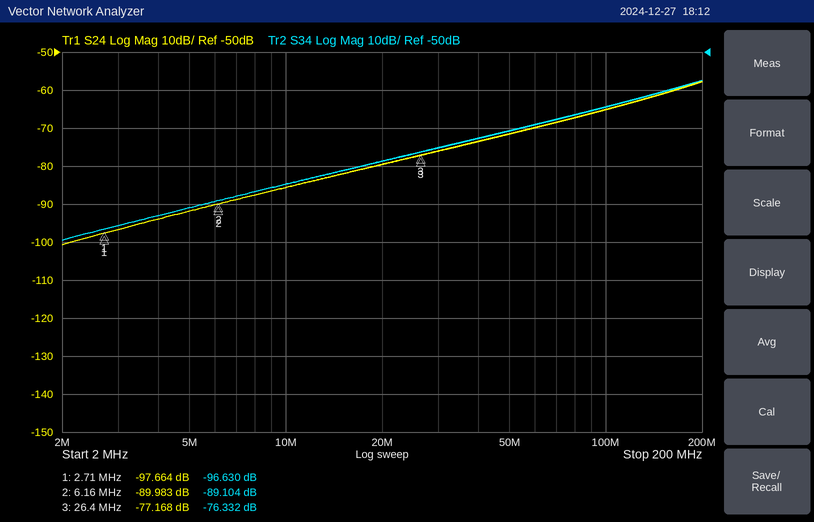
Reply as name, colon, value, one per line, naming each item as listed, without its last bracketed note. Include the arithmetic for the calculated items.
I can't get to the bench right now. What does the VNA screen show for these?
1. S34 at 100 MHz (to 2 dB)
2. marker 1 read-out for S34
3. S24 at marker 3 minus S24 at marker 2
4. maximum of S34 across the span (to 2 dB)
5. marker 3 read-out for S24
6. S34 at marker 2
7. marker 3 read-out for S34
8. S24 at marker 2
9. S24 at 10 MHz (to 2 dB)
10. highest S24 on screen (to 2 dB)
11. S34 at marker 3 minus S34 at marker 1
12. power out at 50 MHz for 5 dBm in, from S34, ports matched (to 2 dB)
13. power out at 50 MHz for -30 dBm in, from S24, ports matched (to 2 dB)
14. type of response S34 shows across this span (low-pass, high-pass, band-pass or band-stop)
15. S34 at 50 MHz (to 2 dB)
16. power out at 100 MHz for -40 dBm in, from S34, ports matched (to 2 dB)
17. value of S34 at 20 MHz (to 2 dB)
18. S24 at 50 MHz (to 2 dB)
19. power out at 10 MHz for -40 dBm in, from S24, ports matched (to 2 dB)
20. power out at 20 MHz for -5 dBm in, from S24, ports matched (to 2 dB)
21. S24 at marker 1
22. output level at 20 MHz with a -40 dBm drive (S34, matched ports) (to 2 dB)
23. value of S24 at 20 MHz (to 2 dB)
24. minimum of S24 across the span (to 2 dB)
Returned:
S34 at 100 MHz: -64 dB
marker 1 read-out for S34: -96.630 dB
S24 at marker 3 minus S24 at marker 2: -77.168 − (-89.983) = 12.815 dB
maximum of S34 across the span: -58 dB
marker 3 read-out for S24: -77.168 dB
S34 at marker 2: -89.104 dB
marker 3 read-out for S34: -76.332 dB
S24 at marker 2: -89.983 dB
S24 at 10 MHz: -86 dB
highest S24 on screen: -58 dB
S34 at marker 3 minus S34 at marker 1: -76.332 − (-96.63) = 20.298 dB
power out at 50 MHz for 5 dBm in, from S34, ports matched: 5 dBm + (-70 dB) = -66 dBm
power out at 50 MHz for -30 dBm in, from S24, ports matched: -30 dBm + (-72 dB) = -102 dBm
type of response S34 shows across this span: high-pass
S34 at 50 MHz: -70 dB
power out at 100 MHz for -40 dBm in, from S34, ports matched: -40 dBm + (-64 dB) = -104 dBm
value of S34 at 20 MHz: -78 dB
S24 at 50 MHz: -72 dB
power out at 10 MHz for -40 dBm in, from S24, ports matched: -40 dBm + (-86 dB) = -126 dBm
power out at 20 MHz for -5 dBm in, from S24, ports matched: -5 dBm + (-80 dB) = -84 dBm
S24 at marker 1: -97.664 dB
output level at 20 MHz with a -40 dBm drive (S34, matched ports): -40 dBm + (-78 dB) = -118 dBm
value of S24 at 20 MHz: -80 dB
minimum of S24 across the span: -100 dB
